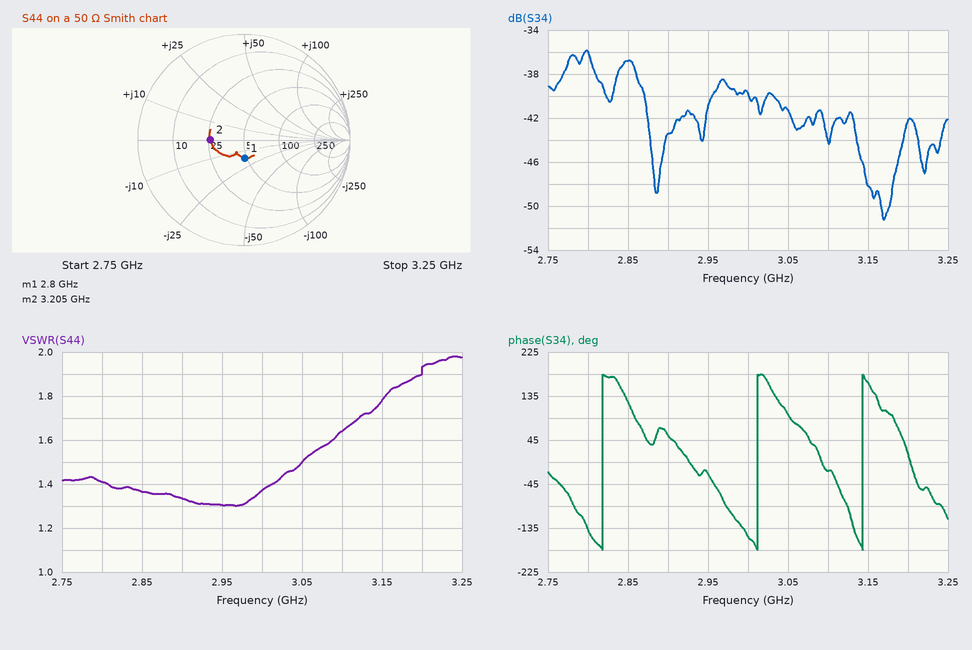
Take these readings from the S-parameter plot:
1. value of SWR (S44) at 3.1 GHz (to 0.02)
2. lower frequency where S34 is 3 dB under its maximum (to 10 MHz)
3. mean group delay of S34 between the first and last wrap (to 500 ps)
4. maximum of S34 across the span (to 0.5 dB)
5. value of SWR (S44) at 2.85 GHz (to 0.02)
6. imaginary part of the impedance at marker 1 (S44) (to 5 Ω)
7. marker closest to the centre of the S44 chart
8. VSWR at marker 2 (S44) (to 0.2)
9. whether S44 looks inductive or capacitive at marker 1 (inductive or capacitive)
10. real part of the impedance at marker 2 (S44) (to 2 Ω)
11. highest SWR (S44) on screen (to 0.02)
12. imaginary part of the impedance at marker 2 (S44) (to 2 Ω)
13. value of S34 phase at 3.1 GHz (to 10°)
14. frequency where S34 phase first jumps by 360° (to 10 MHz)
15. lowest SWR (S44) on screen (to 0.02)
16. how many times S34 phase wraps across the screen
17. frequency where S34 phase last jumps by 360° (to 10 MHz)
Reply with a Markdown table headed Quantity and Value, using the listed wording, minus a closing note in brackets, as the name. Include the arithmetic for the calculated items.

| Quantity | Value |
|---|---|
| value of SWR (S44) at 3.1 GHz | 1.64 |
| lower frequency where S34 is 3 dB under its maximum | 2.76 GHz |
| mean group delay of S34 between the first and last wrap | 2 cycles / (3.14 GHz − 2.82 GHz) ≈ 6.25 ns, so 6.0 ns to the nearest 500 ps |
| maximum of S34 across the span | -36.0 dB |
| value of SWR (S44) at 2.85 GHz | 1.36 |
| imaginary part of the impedance at marker 1 (S44) | -15 Ω |
| marker closest to the centre of the S44 chart | marker 1 |
| VSWR at marker 2 (S44) | 2.0 |
| whether S44 looks inductive or capacitive at marker 1 | capacitive |
| real part of the impedance at marker 2 (S44) | 26 Ω |
| highest SWR (S44) on screen | 1.98 |
| imaginary part of the impedance at marker 2 (S44) | 0 Ω |
| value of S34 phase at 3.1 GHz | -20° |
| frequency where S34 phase first jumps by 360° | 2.82 GHz |
| lowest SWR (S44) on screen | 1.30 |
| how many times S34 phase wraps across the screen | 3 |
| frequency where S34 phase last jumps by 360° | 3.14 GHz |
